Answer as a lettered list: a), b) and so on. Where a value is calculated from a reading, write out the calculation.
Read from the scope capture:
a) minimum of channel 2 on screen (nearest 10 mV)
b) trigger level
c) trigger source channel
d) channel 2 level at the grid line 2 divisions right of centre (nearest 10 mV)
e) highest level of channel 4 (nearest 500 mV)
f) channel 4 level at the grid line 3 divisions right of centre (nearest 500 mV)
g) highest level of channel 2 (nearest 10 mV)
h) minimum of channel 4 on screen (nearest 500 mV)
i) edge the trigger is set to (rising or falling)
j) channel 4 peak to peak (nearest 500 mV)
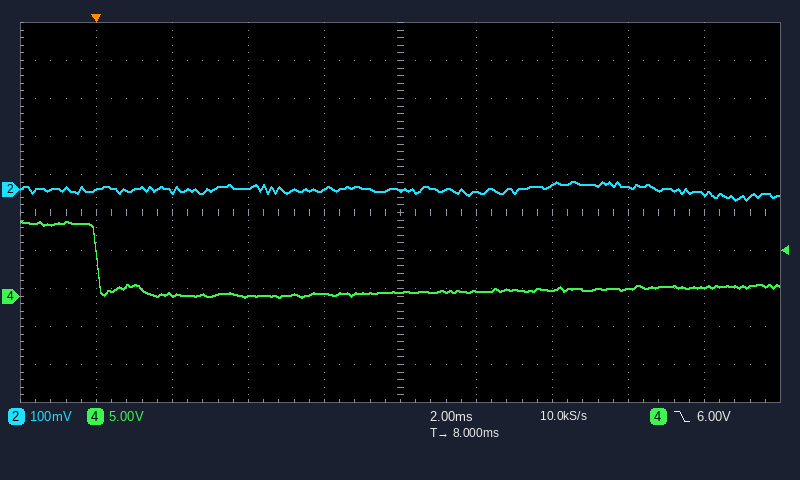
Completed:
a) -30 mV
b) 6.00 V
c) channel 4
d) 10 mV
e) 10.0 V
f) 1.0 V
g) 20 mV
h) 0.0 V
i) falling
j) 10.0 V − (0.0 V) = 10.0 V
